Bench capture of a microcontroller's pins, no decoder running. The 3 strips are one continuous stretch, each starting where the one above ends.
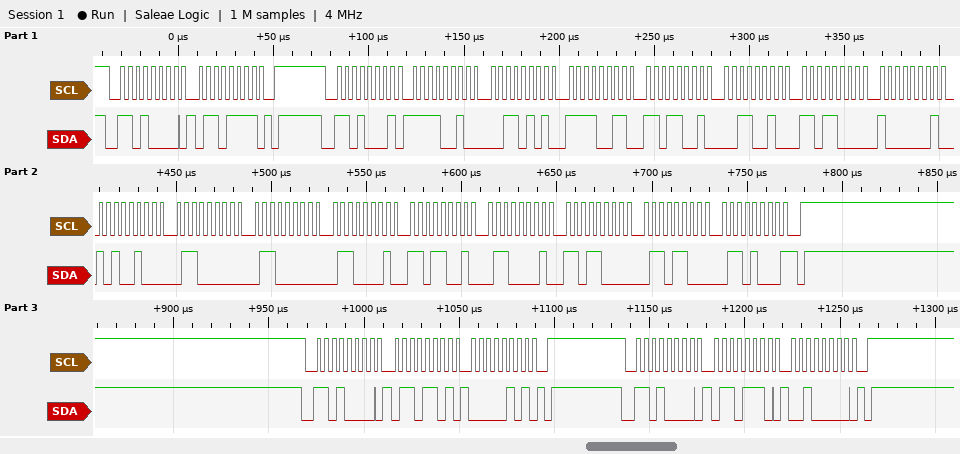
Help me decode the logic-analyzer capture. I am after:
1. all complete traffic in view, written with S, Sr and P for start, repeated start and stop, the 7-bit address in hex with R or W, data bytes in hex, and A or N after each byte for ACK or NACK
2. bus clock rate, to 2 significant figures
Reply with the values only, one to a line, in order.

S 68W A 6F A P S 68R A F2 A 35 A F3 A D9 A 32 A D8 A 81 A A4 A 60 A 60 A 61 A D9 A 61 A D8 A 6C A 68 N P S 68W A 6D A 05 A P S 68W A 6E A 20 A P
250 kHz
